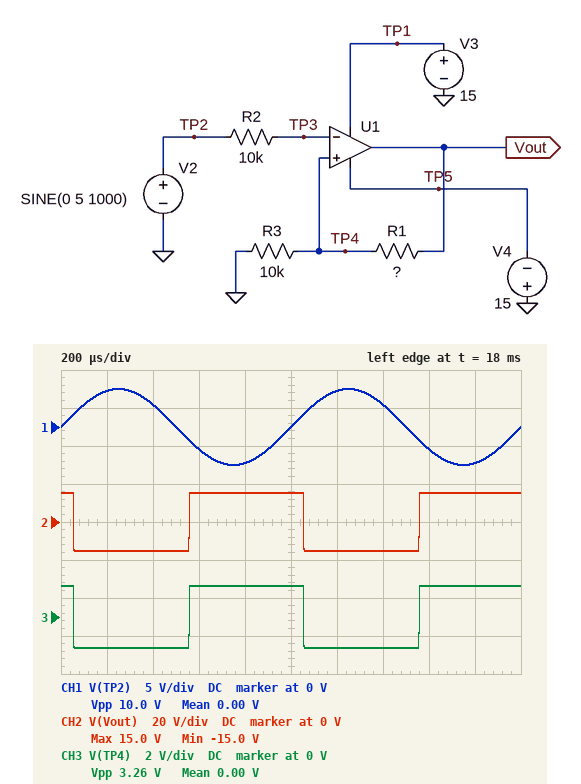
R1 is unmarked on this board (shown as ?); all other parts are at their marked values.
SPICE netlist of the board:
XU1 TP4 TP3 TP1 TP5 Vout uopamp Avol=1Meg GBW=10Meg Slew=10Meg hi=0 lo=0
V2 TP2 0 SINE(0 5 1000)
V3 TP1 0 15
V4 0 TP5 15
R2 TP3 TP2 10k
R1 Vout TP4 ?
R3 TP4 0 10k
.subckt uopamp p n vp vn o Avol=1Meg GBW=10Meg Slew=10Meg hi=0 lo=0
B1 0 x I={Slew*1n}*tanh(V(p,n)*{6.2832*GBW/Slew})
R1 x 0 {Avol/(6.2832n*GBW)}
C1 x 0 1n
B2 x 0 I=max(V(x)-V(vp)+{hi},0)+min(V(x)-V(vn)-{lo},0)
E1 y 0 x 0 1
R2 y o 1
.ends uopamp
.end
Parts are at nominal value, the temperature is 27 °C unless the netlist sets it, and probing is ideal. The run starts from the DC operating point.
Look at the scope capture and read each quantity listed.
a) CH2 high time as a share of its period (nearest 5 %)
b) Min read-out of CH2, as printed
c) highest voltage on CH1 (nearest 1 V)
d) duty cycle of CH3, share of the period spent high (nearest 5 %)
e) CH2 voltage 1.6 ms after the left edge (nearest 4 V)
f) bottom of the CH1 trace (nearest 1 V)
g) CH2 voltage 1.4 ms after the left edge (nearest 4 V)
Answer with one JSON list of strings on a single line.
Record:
["50 %", "-15.0 V", "5 V", "50 %", "16 V", "-5 V", "-16 V"]
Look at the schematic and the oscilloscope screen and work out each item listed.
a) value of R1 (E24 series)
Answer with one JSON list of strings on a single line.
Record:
["82 kΩ"]
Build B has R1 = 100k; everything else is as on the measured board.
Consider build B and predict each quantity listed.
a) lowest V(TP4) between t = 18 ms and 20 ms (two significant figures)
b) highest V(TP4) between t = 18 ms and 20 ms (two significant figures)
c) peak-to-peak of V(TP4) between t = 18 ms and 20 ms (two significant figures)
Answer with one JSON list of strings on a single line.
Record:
["-1.4 V", "1.4 V", "2.7 V"]
